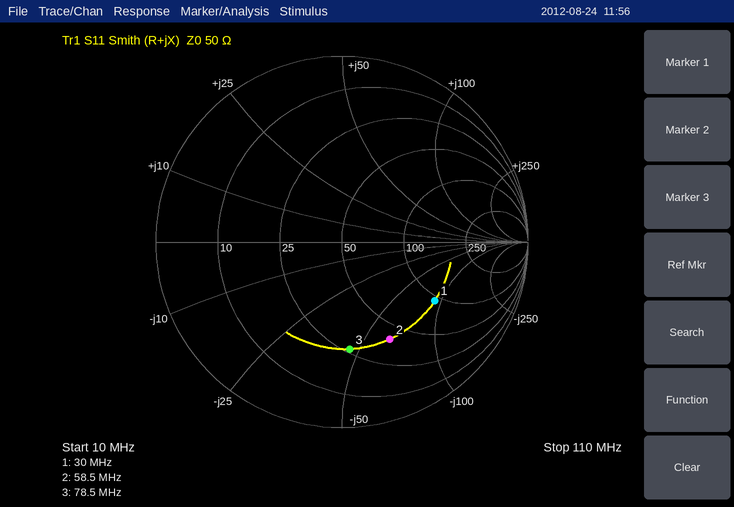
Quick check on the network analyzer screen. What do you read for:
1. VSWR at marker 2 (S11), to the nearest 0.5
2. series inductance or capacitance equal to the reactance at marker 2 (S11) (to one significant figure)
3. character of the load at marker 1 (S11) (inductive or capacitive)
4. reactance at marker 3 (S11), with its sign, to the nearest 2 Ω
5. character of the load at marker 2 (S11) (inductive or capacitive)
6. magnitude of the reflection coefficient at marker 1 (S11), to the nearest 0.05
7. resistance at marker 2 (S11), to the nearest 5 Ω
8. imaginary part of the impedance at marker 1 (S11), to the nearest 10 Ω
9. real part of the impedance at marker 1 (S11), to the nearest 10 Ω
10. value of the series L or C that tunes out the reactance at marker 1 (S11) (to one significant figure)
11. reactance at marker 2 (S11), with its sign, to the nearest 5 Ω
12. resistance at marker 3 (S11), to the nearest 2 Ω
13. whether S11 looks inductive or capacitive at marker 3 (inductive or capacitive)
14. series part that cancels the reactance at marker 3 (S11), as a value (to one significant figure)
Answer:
4.0
40 pF
capacitive
-46 Ω
capacitive
0.60
40 Ω
-90 Ω
90 Ω
500 nH
-65 Ω
26 Ω
capacitive
90 nH
